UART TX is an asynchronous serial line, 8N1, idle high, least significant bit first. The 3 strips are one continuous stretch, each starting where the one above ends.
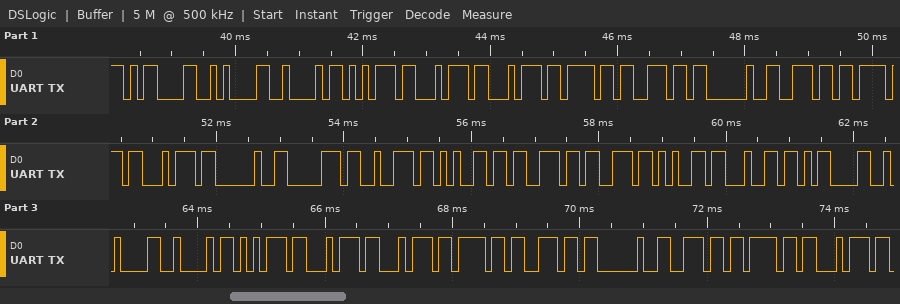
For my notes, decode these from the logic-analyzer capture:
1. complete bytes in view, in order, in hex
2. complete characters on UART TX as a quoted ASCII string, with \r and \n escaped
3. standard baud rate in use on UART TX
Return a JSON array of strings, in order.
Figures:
["0D 0A 42 75 74 74 6F 6E 20 6E 6F 74 20 70 72 65 73 73 65 64 0D 0A 42 75 74 74 6F 6E 20 6E 6F 74", "\"\\r\\nButton not pressed\\r\\nButton not\"", "9600 baud"]
